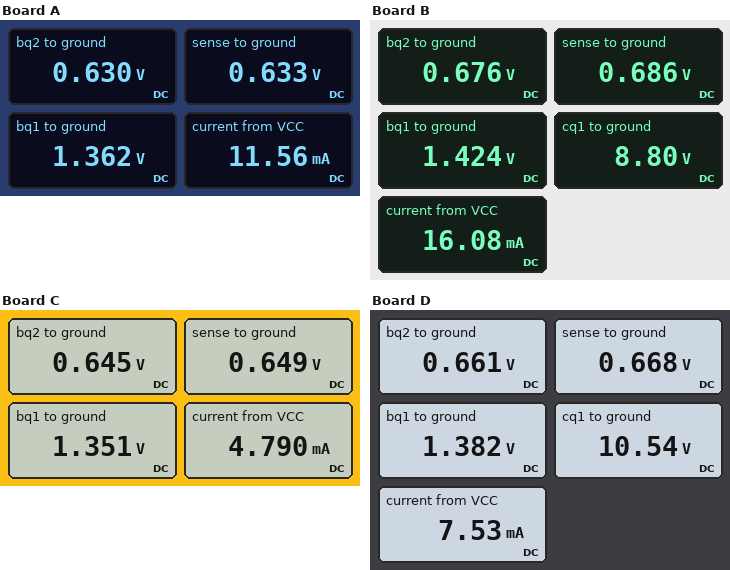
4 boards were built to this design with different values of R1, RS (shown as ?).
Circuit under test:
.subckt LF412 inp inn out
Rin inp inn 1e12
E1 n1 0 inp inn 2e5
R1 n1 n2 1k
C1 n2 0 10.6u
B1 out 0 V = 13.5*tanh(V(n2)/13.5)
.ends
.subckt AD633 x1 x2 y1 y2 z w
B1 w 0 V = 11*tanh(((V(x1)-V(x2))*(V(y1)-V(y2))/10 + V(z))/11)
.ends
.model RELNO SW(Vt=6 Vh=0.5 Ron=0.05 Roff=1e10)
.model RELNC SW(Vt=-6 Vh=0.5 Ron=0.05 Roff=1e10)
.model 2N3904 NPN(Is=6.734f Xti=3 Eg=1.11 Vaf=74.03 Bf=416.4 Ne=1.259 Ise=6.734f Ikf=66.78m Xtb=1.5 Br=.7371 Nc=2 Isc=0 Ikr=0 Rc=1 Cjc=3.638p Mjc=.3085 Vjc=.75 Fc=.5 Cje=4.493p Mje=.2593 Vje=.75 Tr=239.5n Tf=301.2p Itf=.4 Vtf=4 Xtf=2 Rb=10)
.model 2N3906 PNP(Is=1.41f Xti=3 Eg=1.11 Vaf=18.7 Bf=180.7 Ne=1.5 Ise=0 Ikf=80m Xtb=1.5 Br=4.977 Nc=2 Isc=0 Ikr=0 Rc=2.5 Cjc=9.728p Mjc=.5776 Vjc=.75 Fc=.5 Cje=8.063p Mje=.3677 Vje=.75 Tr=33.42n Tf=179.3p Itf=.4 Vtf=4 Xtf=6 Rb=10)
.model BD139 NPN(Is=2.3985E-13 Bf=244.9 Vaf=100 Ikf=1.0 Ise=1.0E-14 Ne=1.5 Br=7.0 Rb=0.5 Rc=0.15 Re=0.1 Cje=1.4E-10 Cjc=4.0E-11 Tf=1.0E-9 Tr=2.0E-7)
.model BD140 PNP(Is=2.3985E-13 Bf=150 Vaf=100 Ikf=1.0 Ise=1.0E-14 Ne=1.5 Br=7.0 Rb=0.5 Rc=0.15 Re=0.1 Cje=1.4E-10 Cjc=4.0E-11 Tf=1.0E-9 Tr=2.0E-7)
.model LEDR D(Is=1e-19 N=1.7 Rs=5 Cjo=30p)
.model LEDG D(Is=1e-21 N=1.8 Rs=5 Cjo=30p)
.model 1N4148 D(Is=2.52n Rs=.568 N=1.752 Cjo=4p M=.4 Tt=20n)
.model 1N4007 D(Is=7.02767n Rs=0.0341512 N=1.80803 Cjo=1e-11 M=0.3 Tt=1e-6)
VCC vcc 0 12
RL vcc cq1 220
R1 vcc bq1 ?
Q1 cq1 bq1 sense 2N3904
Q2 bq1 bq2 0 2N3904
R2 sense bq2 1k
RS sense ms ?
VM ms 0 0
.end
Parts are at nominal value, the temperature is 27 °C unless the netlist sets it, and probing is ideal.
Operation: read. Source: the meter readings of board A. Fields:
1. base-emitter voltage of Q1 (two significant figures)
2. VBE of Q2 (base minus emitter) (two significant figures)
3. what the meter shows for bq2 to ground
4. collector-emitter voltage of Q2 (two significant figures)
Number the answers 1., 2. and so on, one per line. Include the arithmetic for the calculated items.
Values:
1. 1.362 V - 633 mV = 730 mV
2. 630 mV = 630 mV
3. 0.630 V
4. 1.362 V = 1.4 V
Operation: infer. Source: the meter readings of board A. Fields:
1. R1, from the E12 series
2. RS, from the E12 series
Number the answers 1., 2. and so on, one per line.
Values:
1. 33 kΩ
2. 56 Ω
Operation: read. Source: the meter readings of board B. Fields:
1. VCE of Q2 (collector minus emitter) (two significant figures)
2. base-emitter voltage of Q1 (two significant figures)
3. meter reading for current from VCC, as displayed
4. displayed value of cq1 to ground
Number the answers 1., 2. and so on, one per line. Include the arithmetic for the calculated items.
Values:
1. 1.424 V = 1.4 V
2. 1.424 V - 686 mV = 740 mV
3. 16.08 mA
4. 8.80 V
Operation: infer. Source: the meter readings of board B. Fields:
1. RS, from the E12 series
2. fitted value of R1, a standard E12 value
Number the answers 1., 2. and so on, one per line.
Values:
1. 47 Ω
2. 6.8 kΩ
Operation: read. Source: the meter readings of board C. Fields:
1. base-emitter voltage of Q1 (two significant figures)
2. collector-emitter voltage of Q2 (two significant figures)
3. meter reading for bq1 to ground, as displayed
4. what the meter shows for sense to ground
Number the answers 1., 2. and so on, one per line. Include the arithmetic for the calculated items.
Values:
1. 1.351 V - 649 mV = 700 mV
2. 1.351 V = 1.4 V
3. 1.351 V
4. 0.649 V
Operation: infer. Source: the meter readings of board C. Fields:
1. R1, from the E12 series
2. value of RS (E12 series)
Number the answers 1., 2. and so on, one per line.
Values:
1. 22 kΩ
2. 150 Ω
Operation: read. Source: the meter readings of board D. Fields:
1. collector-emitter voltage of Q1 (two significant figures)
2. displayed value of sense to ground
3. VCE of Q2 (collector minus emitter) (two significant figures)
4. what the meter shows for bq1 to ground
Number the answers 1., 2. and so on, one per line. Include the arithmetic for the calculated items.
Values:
1. 10.54 V - 668 mV = 9.9 V
2. 0.668 V
3. 1.382 V = 1.4 V
4. 1.382 V
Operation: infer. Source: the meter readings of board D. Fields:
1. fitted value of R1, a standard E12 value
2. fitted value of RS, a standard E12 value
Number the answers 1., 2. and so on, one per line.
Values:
1. 12 kΩ
2. 100 Ω
